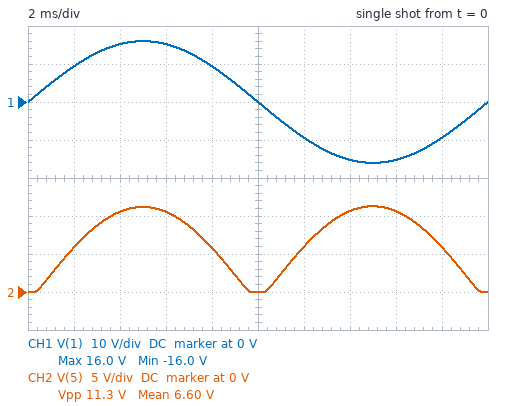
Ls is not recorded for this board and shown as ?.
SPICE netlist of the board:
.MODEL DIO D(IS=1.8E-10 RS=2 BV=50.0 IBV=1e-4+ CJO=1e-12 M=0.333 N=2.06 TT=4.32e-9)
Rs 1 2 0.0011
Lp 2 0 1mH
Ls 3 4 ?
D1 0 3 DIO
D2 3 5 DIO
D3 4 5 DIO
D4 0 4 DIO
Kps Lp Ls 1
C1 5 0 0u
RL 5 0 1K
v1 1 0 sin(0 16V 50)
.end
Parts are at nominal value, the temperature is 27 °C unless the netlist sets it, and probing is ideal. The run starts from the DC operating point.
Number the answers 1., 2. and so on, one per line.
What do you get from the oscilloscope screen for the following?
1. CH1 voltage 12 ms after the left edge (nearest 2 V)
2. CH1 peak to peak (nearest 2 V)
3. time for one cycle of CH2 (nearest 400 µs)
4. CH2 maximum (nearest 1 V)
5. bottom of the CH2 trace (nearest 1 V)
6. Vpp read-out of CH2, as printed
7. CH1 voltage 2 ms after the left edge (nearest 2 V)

1. -10 V
2. 32 V
3. 10.0 ms
4. 11 V
5. 0 V
6. 11.3 V
7. 10 V
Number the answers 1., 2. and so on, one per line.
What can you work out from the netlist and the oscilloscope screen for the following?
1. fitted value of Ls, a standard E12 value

1. 680 µH
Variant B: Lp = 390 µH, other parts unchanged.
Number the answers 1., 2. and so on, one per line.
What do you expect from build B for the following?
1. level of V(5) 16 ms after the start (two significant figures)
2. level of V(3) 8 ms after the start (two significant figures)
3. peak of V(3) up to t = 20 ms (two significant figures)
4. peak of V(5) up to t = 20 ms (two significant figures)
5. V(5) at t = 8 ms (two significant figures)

1. 18 V
2. 11 V
3. 20 V
4. 19 V
5. 10 V
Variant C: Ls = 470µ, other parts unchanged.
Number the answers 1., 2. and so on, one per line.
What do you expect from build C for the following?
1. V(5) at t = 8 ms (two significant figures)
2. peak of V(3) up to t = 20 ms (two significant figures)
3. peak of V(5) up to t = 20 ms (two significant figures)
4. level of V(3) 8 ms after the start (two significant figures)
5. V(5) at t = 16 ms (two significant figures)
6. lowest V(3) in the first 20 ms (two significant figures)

1. 4.5 V
2. 10 V
3. 9.1 V
4. 5.5 V
5. 8.5 V
6. -960 mV
